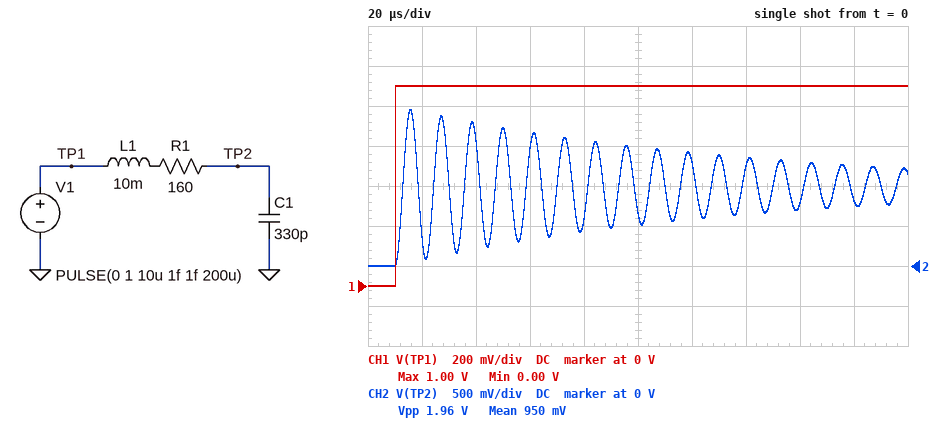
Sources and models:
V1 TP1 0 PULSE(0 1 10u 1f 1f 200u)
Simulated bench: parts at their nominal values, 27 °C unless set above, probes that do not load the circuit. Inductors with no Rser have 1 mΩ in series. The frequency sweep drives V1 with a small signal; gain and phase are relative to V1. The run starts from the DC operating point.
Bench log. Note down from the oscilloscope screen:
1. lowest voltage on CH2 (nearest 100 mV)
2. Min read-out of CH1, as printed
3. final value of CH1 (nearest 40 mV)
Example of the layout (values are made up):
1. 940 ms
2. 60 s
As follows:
1. 0 V
2. 0.00 V
3. 1.00 V
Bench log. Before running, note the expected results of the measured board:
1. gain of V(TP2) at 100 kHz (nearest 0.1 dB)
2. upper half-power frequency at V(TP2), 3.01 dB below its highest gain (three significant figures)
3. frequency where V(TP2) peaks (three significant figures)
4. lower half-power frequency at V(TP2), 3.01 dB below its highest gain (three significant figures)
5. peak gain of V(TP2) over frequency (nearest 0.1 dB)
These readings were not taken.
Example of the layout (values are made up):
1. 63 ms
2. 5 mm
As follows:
1. 10.3 dB
2. 88.9 kHz
3. 87.6 kHz
4. 86.3 kHz
5. 30.7 dB
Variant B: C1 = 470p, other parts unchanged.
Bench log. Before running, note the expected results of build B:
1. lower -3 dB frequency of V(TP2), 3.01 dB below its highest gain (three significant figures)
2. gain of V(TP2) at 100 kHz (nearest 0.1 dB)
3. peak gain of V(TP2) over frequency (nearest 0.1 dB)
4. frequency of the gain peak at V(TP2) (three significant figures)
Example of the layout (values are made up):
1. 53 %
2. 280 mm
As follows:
1. 72.1 kHz
2. 1.3 dB
3. 29.2 dB
4. 73.4 kHz
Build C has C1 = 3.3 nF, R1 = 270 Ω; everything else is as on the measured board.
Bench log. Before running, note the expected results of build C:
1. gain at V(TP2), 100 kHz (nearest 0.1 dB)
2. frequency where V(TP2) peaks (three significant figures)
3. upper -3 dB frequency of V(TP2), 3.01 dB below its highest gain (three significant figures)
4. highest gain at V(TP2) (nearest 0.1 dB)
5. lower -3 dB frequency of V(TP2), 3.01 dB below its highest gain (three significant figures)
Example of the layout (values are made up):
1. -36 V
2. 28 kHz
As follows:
1. -21.6 dB
2. 27.5 kHz
3. 29.6 kHz
4. 16.2 dB
5. 25.3 kHz
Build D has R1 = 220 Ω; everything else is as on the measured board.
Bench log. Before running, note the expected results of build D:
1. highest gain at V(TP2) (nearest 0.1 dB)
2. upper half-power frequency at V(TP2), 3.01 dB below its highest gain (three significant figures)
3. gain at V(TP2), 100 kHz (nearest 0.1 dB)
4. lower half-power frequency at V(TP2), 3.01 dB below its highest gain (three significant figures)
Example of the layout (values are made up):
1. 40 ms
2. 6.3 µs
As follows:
1. 28.0 dB
2. 89.3 kHz
3. 10.3 dB
4. 85.8 kHz
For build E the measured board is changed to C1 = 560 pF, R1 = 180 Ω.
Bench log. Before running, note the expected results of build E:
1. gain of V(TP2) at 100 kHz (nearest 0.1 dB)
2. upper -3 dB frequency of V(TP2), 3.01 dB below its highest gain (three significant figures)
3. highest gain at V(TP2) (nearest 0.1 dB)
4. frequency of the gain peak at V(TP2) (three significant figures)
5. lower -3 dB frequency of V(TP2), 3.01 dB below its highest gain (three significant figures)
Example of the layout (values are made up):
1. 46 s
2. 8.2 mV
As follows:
1. -1.7 dB
2. 68.6 kHz
3. 27.4 dB
4. 67.2 kHz
5. 65.8 kHz
